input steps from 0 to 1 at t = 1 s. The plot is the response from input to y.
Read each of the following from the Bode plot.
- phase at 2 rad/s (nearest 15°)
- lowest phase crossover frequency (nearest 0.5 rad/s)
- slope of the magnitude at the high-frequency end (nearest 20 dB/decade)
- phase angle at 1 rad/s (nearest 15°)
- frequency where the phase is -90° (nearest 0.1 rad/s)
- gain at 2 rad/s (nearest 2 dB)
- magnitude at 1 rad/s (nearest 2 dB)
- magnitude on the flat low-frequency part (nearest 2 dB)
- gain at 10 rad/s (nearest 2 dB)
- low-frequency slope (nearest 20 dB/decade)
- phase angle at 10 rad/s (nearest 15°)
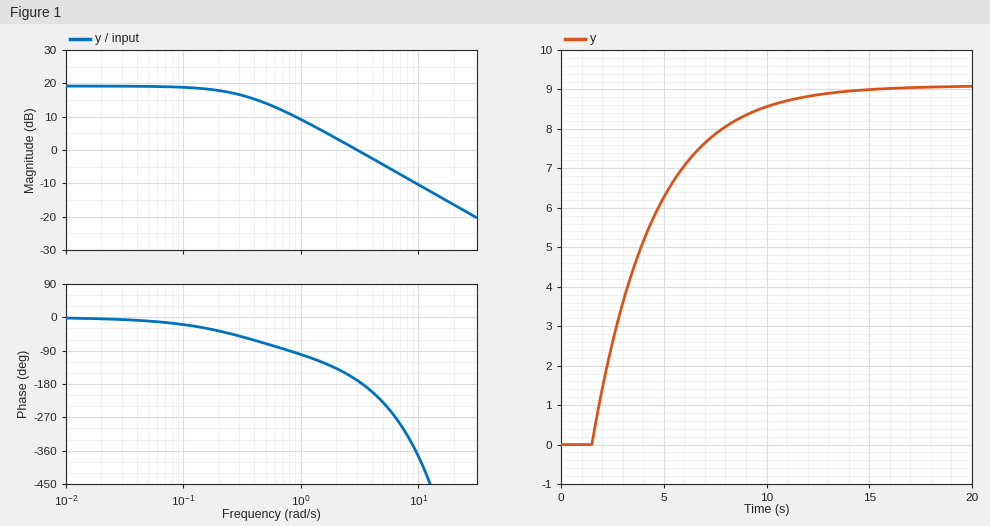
-135°
3.5 rad/s
-20 dB/decade
-105°
0.8 rad/s
4 dB
10 dB
20 dB
-10 dB
0 dB/decade
-375°
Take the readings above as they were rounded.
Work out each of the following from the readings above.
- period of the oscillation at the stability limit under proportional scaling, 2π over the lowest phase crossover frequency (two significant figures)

1.8 s
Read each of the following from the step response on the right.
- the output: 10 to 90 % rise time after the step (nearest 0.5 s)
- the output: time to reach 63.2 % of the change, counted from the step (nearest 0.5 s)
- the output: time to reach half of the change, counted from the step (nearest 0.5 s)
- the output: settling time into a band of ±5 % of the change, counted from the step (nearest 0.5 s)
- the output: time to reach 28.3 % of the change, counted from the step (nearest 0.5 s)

6.5 s
3.5 s
2.5 s
9.5 s
1.5 s
